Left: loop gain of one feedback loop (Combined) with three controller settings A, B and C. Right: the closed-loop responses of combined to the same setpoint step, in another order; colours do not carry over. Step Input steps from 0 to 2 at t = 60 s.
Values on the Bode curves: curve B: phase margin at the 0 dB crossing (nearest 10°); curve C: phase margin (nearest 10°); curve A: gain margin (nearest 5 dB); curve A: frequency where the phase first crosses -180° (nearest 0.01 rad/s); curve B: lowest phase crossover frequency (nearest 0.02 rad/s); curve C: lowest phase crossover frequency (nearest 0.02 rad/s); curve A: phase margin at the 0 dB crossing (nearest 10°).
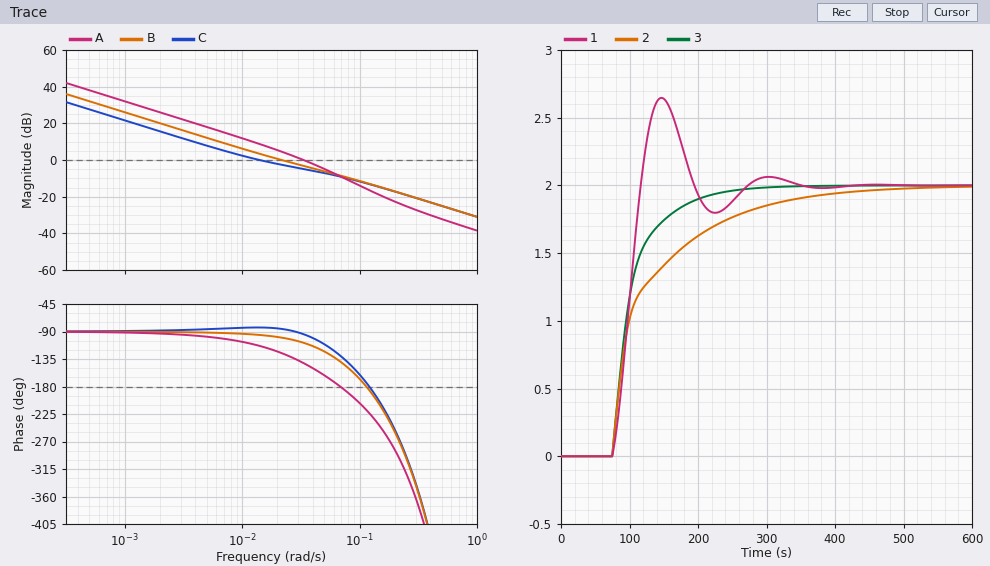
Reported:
80°
100°
10 dB
0.07 rad/s
0.12 rad/s
0.12 rad/s
40°
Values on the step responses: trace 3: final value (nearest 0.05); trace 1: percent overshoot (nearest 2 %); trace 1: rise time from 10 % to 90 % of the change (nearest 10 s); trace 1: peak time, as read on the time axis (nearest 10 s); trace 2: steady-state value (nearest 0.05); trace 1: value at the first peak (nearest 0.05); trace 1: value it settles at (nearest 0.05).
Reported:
2.00
32 %
30 s
150 s
2.00
2.65
2.00
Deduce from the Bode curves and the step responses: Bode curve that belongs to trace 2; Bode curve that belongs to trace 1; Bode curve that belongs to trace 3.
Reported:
C
A
B
